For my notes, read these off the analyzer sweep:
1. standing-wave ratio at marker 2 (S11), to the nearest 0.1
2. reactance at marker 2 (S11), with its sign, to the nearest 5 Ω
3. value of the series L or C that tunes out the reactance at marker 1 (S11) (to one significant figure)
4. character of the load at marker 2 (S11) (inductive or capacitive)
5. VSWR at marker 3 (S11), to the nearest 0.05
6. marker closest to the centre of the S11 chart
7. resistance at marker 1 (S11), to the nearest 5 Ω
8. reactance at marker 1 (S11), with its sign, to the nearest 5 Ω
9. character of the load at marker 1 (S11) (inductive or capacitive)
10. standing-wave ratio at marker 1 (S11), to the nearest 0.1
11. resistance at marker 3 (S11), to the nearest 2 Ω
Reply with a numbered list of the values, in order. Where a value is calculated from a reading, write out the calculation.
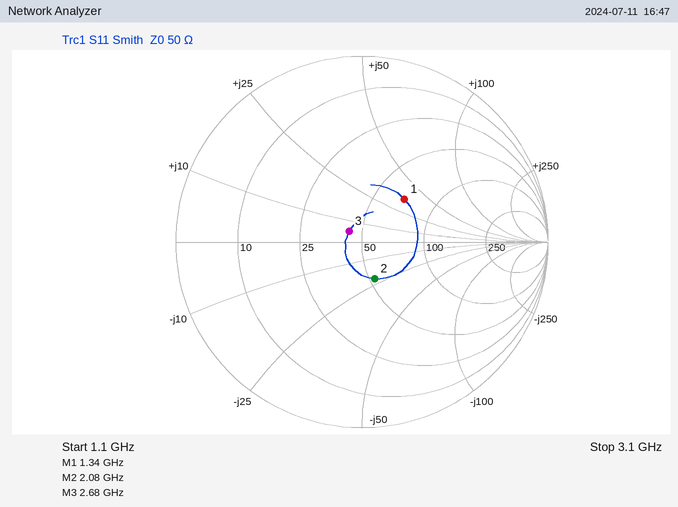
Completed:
1. 1.5
2. -20 Ω
3. C = 1/(2π × 1.34 GHz × 35 Ω) ≈ 3 pF
4. capacitive
5. 1.20
6. marker 3
7. 70 Ω
8. +35 Ω
9. inductive
10. 2.0
11. 44 Ω
